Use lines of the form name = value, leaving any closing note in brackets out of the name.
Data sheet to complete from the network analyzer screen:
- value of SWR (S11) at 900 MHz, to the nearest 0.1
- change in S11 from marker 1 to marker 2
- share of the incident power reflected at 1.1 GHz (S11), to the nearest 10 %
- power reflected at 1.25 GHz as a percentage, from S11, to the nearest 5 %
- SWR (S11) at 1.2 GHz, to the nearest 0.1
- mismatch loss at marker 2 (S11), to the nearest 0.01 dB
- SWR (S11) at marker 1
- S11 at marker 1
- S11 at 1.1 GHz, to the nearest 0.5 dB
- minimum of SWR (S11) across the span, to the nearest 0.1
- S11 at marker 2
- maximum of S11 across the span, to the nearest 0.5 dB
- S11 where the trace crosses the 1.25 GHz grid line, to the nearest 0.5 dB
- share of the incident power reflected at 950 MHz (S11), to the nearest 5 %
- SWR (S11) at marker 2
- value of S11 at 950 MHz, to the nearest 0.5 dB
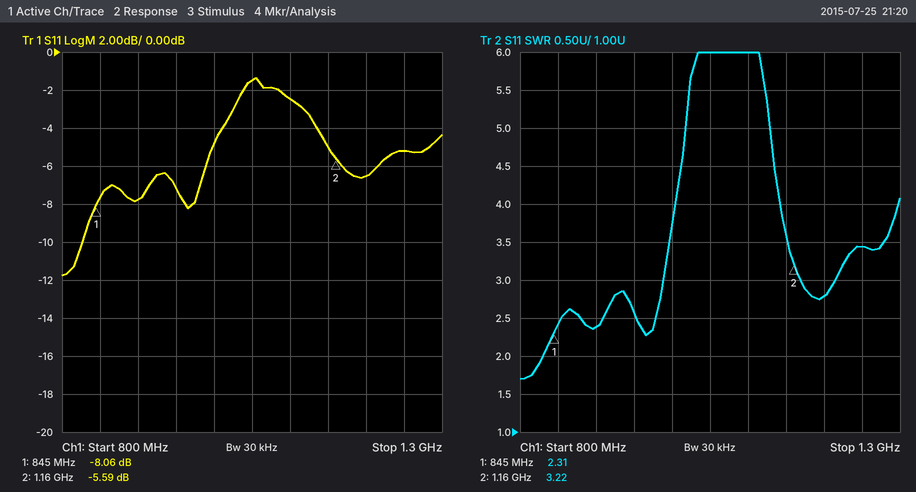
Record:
value of SWR (S11) at 900 MHz, to the nearest 0.1 = 2.4
change in S11 from marker 1 to marker 2 = 2.47 dB
share of the incident power reflected at 1.1 GHz (S11), to the nearest 10 % = 60 %
power reflected at 1.25 GHz as a percentage, from S11, to the nearest 5 % = 30 %
SWR (S11) at 1.2 GHz, to the nearest 0.1 = 2.8
mismatch loss at marker 2 (S11), to the nearest 0.01 dB = 1.40 dB
SWR (S11) at marker 1 = 2.31
S11 at marker 1 = -8.06 dB
S11 at 1.1 GHz, to the nearest 0.5 dB = -2.5 dB
minimum of SWR (S11) across the span, to the nearest 0.1 = 1.7
S11 at marker 2 = -5.59 dB
maximum of S11 across the span, to the nearest 0.5 dB = -1.5 dB
S11 where the trace crosses the 1.25 GHz grid line, to the nearest 0.5 dB = -5.0 dB
share of the incident power reflected at 950 MHz (S11), to the nearest 5 % = 20 %
SWR (S11) at marker 2 = 3.22
value of S11 at 950 MHz, to the nearest 0.5 dB = -7.0 dB
